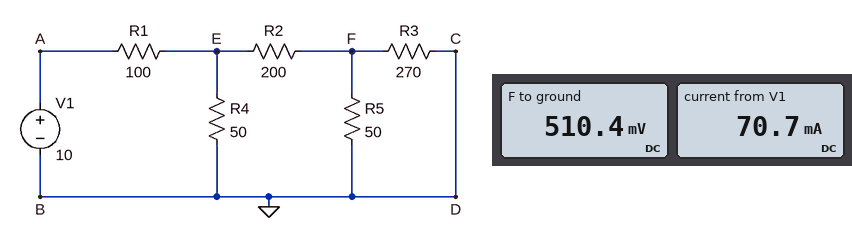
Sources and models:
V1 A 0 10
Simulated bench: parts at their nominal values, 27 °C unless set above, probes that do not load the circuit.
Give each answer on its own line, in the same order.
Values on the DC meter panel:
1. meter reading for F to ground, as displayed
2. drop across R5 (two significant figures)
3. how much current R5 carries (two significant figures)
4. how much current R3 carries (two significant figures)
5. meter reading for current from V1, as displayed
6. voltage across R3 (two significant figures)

510.4 mV
510 mV
10 mA
1.9 mA
70.7 mA
510 mV
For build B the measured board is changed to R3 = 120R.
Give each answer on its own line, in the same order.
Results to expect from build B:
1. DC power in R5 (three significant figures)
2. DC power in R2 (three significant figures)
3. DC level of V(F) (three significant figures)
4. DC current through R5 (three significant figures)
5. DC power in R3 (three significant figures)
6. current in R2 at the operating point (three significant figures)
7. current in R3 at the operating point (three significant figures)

3.84 mW
30.8 mW
438 mV
8.76 mA
1.60 mW
12.4 mA
3.65 mA
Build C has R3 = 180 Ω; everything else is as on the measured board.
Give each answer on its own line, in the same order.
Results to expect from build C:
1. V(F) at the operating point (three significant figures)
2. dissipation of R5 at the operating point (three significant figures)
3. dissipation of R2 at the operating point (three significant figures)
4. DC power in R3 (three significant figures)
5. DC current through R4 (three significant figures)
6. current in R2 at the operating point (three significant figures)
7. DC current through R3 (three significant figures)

479 mV
4.58 mW
29.9 mW
1.27 mW
58.5 mA
12.2 mA
2.66 mA
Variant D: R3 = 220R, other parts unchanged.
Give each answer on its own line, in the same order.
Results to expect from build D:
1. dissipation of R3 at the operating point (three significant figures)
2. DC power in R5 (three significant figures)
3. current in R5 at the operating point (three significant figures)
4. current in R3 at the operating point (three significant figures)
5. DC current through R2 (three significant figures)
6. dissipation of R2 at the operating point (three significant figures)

1.12 mW
4.91 mW
9.91 mA
2.25 mA
12.2 mA
29.6 mW
